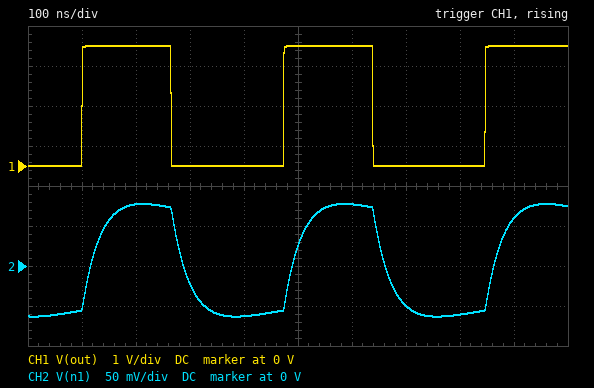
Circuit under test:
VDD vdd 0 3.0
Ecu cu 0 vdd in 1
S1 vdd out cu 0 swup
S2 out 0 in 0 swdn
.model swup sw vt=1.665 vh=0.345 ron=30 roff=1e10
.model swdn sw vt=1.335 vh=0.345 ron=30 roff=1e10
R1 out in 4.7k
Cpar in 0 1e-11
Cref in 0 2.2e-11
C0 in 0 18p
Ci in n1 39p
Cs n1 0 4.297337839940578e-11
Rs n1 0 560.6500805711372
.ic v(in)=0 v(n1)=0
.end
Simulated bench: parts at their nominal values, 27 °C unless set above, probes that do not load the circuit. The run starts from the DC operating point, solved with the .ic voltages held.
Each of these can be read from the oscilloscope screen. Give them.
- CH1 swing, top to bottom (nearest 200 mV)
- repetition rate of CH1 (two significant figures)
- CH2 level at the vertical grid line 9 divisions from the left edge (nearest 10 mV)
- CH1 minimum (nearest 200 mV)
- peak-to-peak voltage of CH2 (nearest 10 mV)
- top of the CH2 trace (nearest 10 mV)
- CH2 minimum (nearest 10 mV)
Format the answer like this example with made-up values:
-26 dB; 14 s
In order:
3.0 V; 2.7 MHz; 60 mV; 0 V; 140 mV; 80 mV; -60 mV
